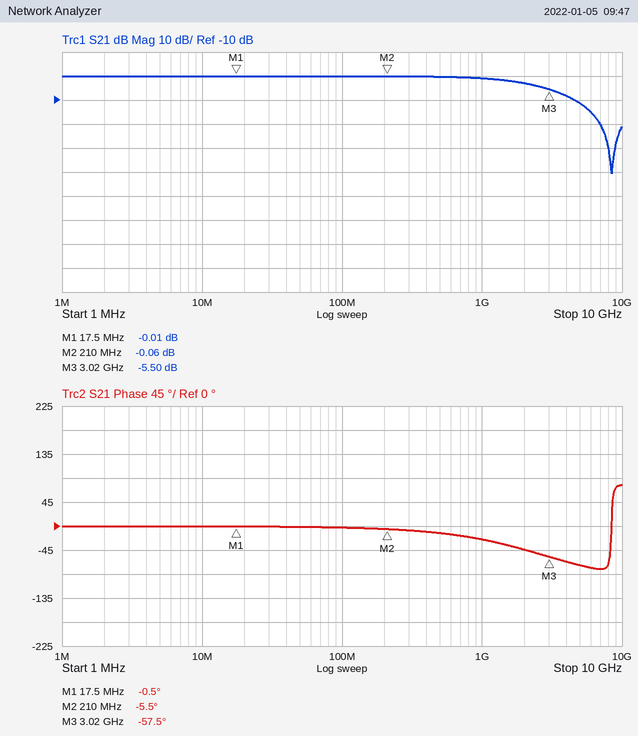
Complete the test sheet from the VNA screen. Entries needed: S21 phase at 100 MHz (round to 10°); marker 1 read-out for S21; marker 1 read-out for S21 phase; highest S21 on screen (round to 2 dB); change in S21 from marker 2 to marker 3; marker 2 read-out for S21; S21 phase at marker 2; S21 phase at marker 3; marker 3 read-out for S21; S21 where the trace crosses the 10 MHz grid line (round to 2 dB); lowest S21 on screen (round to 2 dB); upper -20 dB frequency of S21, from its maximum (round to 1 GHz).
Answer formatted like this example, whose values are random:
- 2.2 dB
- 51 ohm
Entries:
- 0°
- -0.01 dB
- -0.5°
- 0 dB
- -5.44 dB
- -0.06 dB
- -5.5°
- -57.5°
- -5.50 dB
- 0 dB
- -40 dB
- 7 GHz
